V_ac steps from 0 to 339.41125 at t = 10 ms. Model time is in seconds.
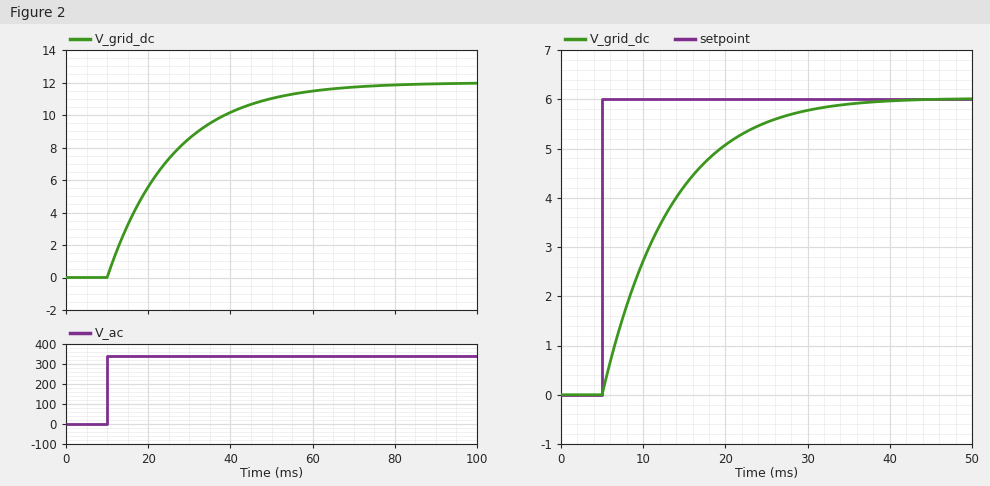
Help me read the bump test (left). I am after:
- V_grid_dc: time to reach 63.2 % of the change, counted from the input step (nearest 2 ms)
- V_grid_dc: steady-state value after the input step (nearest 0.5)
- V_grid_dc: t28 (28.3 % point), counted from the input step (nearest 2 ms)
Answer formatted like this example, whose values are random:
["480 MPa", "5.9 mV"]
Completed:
["16 ms", "12.0", "6 ms"]
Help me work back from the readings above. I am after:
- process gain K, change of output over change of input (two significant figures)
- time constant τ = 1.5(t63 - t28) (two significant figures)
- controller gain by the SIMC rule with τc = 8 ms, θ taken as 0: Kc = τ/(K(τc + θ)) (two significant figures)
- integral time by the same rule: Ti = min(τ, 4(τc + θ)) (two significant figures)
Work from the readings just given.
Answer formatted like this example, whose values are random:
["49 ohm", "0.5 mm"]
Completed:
["0.035", "15 ms", "54", "15 ms"]
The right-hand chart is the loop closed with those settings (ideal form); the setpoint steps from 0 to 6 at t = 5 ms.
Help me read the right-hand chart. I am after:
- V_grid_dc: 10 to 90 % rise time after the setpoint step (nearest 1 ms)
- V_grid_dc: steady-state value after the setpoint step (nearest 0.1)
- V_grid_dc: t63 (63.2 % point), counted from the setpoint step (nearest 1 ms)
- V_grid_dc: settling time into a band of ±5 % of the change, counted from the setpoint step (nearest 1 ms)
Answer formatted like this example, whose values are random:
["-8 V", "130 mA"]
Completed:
["17 ms", "6.0", "8 ms", "23 ms"]
